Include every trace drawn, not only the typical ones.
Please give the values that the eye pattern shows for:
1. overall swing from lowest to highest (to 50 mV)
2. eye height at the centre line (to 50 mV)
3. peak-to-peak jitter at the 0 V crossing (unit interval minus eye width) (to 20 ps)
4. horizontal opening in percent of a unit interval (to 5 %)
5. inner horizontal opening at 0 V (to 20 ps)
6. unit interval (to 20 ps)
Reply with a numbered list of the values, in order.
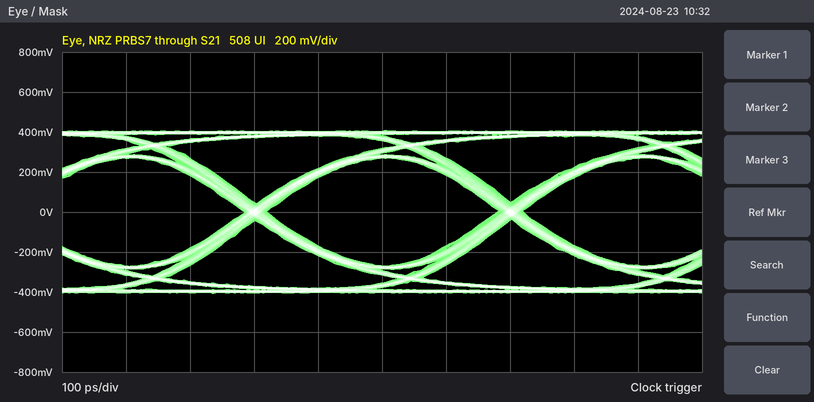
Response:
1. 800 mV
2. 550 mV
3. 40 ps
4. 90 %
5. 360 ps
6. 400 ps
